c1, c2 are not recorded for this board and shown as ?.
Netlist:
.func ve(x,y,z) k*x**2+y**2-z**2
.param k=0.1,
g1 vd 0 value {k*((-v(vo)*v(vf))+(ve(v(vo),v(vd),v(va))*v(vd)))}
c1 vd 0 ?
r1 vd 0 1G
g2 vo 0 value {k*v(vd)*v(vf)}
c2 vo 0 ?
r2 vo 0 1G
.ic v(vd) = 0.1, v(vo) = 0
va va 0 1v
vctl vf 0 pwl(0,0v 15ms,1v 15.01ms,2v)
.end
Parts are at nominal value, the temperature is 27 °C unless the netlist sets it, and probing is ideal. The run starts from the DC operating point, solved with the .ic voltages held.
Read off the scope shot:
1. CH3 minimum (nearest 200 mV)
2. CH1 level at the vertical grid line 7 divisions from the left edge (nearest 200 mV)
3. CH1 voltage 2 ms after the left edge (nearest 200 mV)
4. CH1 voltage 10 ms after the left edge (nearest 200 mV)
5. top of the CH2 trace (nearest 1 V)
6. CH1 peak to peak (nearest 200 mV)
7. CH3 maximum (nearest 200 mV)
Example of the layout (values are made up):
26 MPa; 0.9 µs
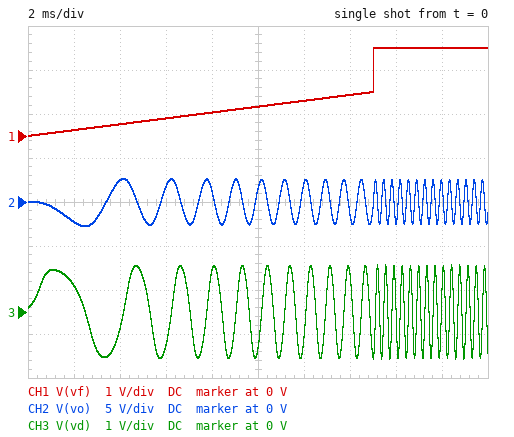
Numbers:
-1.0 V; 1.0 V; 200 mV; 600 mV; 3 V; 2.0 V; 1.0 V
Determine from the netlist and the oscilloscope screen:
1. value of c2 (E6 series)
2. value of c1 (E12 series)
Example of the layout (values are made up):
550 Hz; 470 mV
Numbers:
4.7 µF; 27 µF
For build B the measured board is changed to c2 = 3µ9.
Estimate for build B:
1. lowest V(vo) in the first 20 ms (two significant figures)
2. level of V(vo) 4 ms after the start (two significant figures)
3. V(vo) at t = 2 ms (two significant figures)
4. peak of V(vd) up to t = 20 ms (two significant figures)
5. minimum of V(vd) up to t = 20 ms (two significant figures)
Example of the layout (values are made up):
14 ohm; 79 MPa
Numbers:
-2.9 V; 2.8 V; -2.6 V; 1.0 V; -1.0 V
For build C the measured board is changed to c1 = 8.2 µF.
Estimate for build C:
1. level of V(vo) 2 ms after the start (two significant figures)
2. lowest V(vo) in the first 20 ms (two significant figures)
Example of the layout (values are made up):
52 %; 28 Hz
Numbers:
-2.2 V; -2.3 V
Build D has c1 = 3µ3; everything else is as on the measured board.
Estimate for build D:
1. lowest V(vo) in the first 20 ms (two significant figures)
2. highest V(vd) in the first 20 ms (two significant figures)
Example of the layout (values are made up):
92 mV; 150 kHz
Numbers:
-2.1 V; 1.2 V
